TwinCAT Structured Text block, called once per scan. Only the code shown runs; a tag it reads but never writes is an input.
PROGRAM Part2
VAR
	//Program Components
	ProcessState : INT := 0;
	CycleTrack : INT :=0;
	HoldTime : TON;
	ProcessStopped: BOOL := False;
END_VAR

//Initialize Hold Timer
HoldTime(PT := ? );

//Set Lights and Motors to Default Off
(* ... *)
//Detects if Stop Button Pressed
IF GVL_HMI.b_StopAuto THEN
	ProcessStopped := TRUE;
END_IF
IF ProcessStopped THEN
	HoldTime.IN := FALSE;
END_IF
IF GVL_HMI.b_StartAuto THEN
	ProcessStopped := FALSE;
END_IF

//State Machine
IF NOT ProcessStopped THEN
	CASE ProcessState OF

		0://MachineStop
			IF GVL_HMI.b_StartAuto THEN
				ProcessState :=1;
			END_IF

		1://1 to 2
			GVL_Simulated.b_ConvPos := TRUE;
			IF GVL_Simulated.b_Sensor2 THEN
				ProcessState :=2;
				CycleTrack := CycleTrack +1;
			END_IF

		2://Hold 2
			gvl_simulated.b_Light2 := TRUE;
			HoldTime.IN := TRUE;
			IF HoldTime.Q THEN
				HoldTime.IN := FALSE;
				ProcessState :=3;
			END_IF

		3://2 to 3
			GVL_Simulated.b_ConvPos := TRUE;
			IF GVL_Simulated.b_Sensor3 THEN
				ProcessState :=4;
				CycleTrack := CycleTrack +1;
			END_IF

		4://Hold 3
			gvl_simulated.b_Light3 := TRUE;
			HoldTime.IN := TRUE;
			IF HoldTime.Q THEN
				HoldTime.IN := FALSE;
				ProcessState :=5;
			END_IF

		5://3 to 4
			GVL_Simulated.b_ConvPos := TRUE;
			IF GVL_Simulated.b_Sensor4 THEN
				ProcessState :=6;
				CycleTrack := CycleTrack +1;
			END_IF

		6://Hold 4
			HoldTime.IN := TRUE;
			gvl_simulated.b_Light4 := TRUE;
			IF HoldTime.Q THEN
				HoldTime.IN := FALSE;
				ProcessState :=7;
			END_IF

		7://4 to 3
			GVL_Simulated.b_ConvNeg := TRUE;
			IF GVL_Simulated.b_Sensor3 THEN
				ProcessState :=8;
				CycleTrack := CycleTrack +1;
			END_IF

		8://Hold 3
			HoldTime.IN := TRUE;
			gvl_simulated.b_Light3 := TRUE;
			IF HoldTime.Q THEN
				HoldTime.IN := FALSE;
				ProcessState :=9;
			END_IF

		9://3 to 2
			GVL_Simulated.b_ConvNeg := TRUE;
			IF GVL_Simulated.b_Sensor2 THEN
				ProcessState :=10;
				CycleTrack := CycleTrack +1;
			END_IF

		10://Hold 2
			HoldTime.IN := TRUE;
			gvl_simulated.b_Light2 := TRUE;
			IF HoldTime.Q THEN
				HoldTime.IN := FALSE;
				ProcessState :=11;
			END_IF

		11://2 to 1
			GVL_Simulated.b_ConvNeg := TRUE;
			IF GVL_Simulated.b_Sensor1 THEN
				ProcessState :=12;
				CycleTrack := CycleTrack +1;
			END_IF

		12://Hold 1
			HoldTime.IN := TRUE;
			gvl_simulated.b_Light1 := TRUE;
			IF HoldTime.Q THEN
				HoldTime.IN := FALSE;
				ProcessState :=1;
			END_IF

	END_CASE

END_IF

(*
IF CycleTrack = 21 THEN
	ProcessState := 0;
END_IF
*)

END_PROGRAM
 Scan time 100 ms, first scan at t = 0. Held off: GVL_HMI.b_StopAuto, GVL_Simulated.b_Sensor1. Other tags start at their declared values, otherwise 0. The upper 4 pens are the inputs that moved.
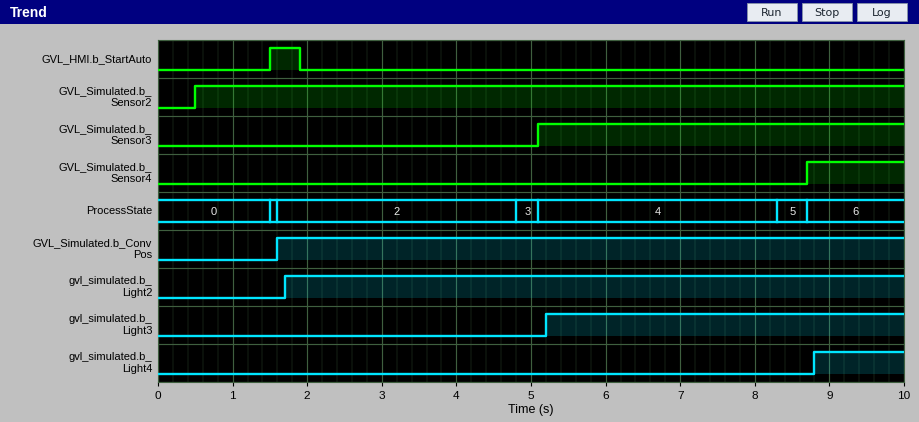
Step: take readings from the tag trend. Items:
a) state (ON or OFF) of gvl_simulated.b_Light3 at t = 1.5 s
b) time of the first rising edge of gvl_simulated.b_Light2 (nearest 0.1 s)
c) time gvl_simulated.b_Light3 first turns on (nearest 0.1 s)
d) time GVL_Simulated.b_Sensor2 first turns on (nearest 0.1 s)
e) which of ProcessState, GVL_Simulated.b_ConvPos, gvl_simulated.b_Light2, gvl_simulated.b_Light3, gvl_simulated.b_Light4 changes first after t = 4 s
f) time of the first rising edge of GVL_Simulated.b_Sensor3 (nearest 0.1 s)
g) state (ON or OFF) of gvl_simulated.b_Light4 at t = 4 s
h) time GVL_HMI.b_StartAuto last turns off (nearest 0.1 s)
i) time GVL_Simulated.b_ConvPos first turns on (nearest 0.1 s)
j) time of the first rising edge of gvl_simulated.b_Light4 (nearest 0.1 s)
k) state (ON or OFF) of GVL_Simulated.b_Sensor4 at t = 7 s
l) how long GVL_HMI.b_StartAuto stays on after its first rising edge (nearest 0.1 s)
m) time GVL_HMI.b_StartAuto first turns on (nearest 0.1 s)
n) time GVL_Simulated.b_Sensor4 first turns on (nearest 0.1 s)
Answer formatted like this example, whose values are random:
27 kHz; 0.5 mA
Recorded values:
OFF; 1.7 s; 5.2 s; 0.5 s; ProcessState; 5.1 s; OFF; 1.9 s; 1.6 s; 8.8 s; OFF; 0.4 s; 1.5 s; 8.7 s
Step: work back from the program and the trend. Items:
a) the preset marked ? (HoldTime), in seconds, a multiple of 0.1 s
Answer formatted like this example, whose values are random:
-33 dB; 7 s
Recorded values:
3.0 s
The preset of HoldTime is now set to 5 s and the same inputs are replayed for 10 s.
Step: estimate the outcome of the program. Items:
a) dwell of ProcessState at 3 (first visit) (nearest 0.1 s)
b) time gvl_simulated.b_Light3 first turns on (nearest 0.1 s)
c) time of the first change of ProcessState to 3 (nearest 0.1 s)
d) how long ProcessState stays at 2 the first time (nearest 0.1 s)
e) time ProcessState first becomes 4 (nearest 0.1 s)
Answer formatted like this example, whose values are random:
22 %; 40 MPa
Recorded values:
0.1 s; 7.0 s; 6.8 s; 5.2 s; 6.9 s
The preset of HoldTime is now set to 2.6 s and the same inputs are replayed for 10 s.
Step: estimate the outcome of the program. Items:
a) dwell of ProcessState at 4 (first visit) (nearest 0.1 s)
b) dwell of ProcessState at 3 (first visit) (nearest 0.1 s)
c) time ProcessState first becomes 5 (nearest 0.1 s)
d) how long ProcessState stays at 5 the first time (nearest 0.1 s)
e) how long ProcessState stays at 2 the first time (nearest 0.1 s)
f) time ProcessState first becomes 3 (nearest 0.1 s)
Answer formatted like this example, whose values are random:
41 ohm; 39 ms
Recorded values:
2.8 s; 0.7 s; 7.9 s; 0.8 s; 2.8 s; 4.4 s
